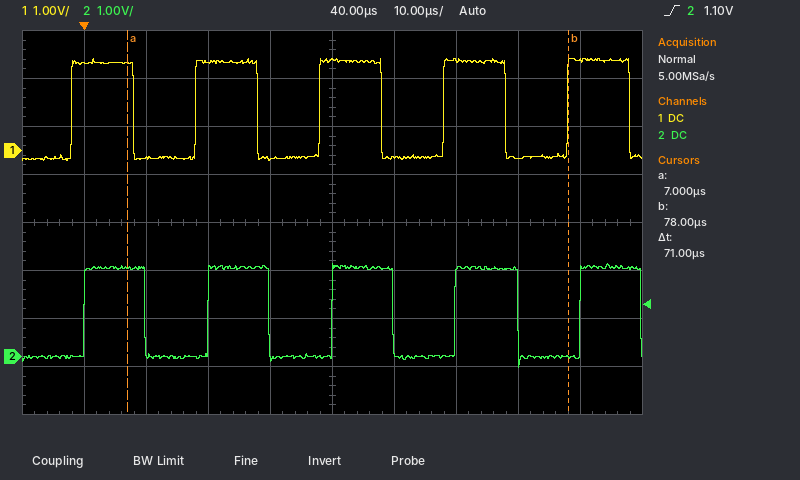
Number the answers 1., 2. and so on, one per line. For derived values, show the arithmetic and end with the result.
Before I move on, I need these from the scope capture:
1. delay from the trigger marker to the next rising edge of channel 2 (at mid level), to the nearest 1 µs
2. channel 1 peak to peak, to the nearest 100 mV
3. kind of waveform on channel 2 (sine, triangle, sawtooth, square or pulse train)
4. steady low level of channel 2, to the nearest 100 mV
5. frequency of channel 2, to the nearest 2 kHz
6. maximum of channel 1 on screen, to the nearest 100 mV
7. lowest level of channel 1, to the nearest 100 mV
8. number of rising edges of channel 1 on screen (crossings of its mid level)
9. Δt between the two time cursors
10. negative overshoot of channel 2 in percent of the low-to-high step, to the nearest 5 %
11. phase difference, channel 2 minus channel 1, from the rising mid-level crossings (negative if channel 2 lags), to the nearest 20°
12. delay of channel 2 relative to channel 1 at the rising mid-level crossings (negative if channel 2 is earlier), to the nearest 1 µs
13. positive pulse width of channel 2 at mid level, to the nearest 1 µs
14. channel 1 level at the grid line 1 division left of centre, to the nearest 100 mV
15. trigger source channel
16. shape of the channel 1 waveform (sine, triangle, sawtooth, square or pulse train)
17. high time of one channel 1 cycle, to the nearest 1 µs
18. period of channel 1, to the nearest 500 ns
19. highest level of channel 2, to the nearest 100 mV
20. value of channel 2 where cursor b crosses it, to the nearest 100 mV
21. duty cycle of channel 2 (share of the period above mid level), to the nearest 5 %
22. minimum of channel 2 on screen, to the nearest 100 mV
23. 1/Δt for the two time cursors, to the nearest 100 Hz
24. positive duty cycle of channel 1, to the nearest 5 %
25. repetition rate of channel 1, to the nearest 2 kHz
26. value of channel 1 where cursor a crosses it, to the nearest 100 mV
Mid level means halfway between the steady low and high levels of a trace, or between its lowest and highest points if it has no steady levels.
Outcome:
1. 20 µs
2. 1.9 V − (-200 mV) = 2.1 V
3. square
4. 0.0 V
5. 1 / 20.0 µs ≈ 50 kHz
6. 1.9 V
7. -200 mV
8. 5
9. 71 µs
10. 10 %
11. −360° × (+2 µs) / 20.0 µs ≈ -36.0°, so -40° to the nearest 20°
12. +2 µs
13. 10 µs
14. -200 mV
15. channel 2
16. square
17. 10 µs
18. 20.0 µs
19. 1.9 V
20. 0.0 V
21. 10 µs / 20.0 µs ≈ 50 %
22. -200 mV
23. 1 / 71 µs ≈ 14.1 kHz
24. 10 µs / 20.0 µs ≈ 50 %
25. 1 / 20.0 µs ≈ 50 kHz
26. 1.8 V
